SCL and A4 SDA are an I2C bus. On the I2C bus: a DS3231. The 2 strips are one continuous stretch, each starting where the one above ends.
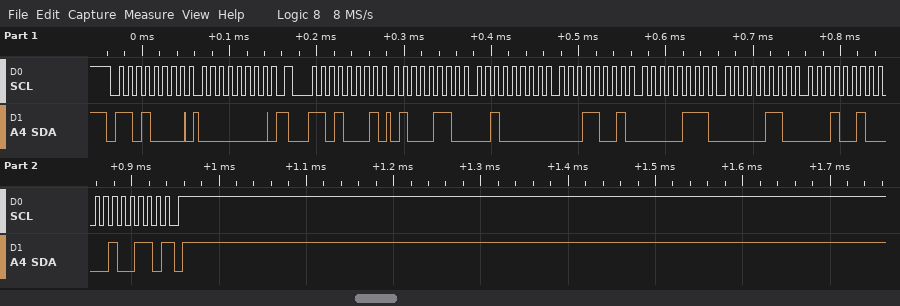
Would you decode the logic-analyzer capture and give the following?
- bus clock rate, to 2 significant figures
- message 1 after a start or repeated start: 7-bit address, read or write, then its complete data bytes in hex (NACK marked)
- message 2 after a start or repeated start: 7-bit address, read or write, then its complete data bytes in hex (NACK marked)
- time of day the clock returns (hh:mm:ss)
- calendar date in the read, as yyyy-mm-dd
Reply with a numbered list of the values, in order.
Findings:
1. 100 kHz
2. 0x68 write: 00
3. 0x68 read: 46 20 19 07 06 12 26 NACK
4. 19:20:46
5. 2026-12-06
